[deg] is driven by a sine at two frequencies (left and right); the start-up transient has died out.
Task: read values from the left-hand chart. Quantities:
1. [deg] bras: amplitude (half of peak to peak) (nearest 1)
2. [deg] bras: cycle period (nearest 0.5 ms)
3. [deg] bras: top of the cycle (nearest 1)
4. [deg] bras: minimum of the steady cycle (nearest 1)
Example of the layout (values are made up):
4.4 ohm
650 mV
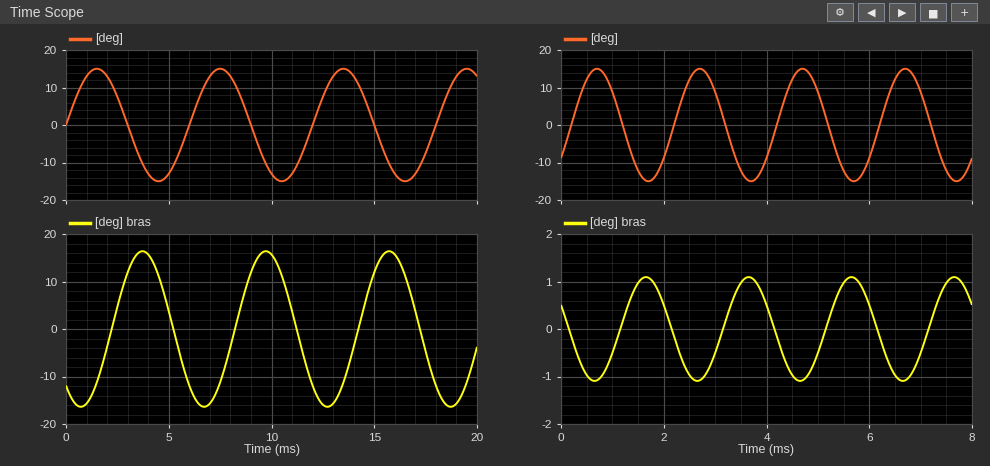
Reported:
16
6.0 ms
16
-16
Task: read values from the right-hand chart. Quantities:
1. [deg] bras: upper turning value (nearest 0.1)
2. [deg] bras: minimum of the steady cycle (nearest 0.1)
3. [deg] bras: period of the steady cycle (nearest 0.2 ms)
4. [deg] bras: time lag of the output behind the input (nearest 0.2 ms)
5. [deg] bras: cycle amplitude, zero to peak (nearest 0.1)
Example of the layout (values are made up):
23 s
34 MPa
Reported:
1.1
-1.1
2.0 ms
1.0 ms
1.1
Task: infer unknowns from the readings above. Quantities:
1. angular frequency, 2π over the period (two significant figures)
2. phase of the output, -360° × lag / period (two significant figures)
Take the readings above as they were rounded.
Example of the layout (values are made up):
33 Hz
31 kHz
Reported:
3.1 rad/ms
-180°
